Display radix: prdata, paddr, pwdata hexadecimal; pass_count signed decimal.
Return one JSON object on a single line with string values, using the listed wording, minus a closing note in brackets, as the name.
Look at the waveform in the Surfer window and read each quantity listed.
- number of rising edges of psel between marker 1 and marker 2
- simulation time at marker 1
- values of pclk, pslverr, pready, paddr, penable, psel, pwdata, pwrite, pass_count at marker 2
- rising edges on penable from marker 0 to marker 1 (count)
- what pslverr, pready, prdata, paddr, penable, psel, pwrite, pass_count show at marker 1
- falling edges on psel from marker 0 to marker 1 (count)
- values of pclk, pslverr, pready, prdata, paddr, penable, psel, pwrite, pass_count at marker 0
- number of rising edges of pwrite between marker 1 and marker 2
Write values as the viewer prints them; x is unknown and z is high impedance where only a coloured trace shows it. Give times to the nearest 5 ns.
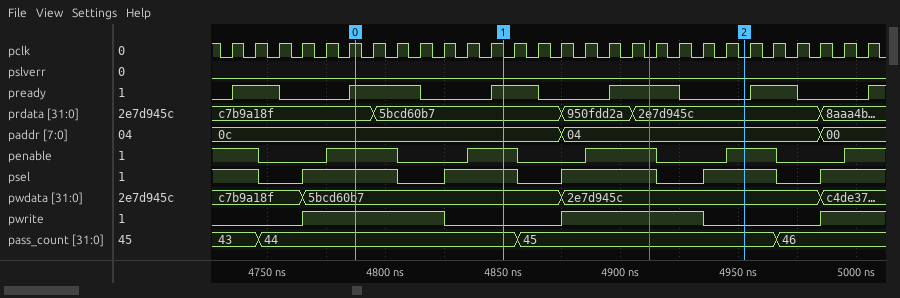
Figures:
{"number of rising edges of psel between marker 1 and marker 2": "2", "simulation time at marker 1": "4850 ns", "values of pclk, pslverr, pready, paddr, penable, psel, pwdata, pwrite, pass_count at marker 2": "pclk=0, pslverr=0, pready=0, paddr=04, penable=1, psel=1, pwdata=2e7d945c, pwrite=0, pass_count=45", "rising edges on penable from marker 0 to marker 1": "1", "what pslverr, pready, prdata, paddr, penable, psel, pwrite, pass_count show at marker 1": "pslverr=0, pready=1, prdata=5bcd60b7, paddr=0c, penable=1, psel=1, pwrite=0, pass_count=44", "falling edges on psel from marker 0 to marker 1": "1", "values of pclk, pslverr, pready, prdata, paddr, penable, psel, pwrite, pass_count at marker 0": "pclk=1, pslverr=0, pready=1, prdata=c7b9a18f, paddr=0c, penable=1, psel=1, pwrite=1, pass_count=44", "number of rising edges of pwrite between marker 1 and marker 2": "1"}
